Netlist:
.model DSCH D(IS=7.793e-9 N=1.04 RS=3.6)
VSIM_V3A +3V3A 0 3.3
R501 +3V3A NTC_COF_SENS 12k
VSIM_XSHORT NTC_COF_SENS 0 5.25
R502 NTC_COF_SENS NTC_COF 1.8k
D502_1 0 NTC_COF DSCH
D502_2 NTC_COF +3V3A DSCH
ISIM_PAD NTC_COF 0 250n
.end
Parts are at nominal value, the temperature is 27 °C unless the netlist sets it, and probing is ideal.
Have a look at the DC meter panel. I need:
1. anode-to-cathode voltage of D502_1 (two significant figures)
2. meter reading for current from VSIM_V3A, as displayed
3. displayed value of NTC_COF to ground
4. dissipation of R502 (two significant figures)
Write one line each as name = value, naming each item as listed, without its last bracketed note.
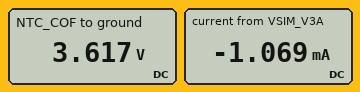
anode-to-cathode voltage of D502_1 = -3.6 V
meter reading for current from VSIM_V3A, as displayed = -1.069 mA
displayed value of NTC_COF to ground = 3.617 V
dissipation of R502 = 1.5 mW
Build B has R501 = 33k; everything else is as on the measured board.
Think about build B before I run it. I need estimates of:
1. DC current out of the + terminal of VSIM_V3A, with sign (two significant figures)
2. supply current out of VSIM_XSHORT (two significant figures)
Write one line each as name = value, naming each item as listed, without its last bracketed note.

DC current out of the + terminal of VSIM_V3A, with sign = -970 µA
supply current out of VSIM_XSHORT = 970 µA
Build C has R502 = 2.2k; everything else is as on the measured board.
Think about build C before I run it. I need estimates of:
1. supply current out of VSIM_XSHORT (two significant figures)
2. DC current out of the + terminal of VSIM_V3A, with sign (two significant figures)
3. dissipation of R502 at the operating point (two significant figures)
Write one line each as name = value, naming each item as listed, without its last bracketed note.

supply current out of VSIM_XSHORT = 910 µA
DC current out of the + terminal of VSIM_V3A, with sign = -910 µA
dissipation of R502 at the operating point = 1.2 mW
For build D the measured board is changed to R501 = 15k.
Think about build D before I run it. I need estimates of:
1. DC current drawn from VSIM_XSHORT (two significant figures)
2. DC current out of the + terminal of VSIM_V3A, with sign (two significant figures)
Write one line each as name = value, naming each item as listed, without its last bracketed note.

DC current drawn from VSIM_XSHORT = 1.0 mA
DC current out of the + terminal of VSIM_V3A, with sign = -1.0 mA
